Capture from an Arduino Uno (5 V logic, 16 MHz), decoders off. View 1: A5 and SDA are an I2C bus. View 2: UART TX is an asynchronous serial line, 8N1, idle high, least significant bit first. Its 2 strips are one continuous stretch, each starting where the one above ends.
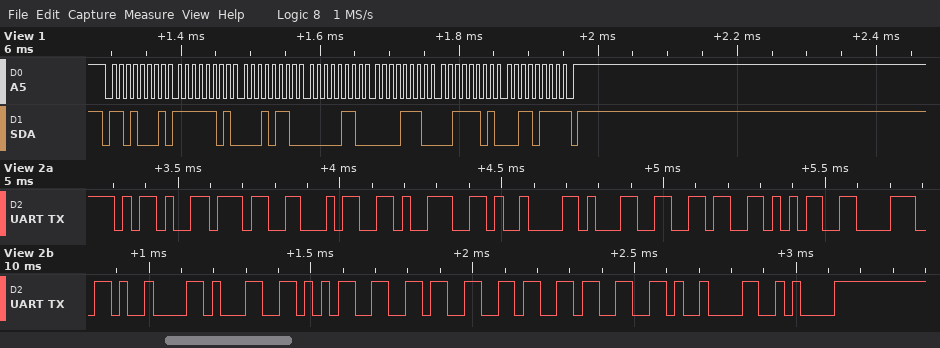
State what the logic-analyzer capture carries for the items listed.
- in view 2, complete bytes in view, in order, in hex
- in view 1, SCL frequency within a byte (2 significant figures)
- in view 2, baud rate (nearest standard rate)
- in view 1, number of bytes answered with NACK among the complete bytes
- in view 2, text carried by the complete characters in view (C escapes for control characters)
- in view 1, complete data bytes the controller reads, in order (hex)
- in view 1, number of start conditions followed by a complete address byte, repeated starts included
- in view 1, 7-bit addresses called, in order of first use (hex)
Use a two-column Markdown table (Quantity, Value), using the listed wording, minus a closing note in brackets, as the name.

| Quantity | Value |
|---|---|
| in view 2, complete bytes in view, in order, in hex | 2D 37 34 39 09 31 36 35 38 09 31 35 36 36 33 09 0A |
| in view 1, SCL frequency within a byte | 100 kHz |
| in view 2, baud rate | 38400 baud |
| in view 1, number of bytes answered with NACK among the complete bytes | 1 |
| in view 2, text carried by the complete characters in view | "-749\t1658\t15663\t\n" |
| in view 1, complete data bytes the controller reads, in order | FD 16 06 0E 3D 37 |
| in view 1, number of start conditions followed by a complete address byte, repeated starts included | 1 |
| in view 1, 7-bit addresses called, in order of first use | 0x68 |
